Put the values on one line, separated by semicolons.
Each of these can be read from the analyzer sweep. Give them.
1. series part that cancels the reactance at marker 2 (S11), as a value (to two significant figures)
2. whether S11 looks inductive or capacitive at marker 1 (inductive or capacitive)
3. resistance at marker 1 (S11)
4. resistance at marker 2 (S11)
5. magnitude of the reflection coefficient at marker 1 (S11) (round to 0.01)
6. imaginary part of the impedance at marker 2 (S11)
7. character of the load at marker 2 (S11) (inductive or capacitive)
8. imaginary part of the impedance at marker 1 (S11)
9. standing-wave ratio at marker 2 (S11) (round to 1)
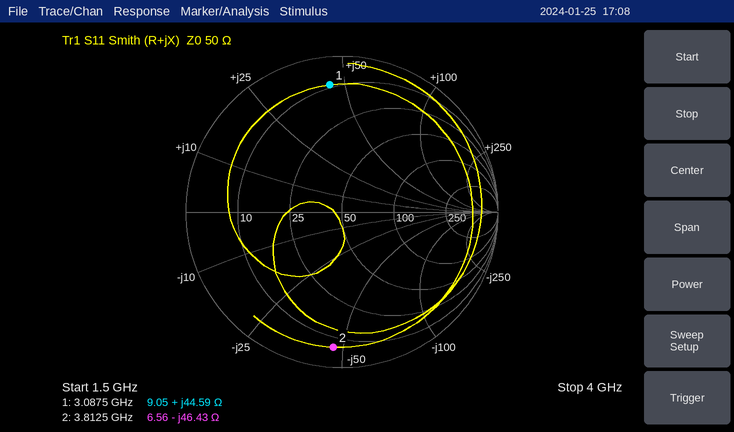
1.9 nH; inductive; 9.05 Ω; 6.56 Ω; 0.82; -46.43 Ω; capacitive; +44.59 Ω; 14
